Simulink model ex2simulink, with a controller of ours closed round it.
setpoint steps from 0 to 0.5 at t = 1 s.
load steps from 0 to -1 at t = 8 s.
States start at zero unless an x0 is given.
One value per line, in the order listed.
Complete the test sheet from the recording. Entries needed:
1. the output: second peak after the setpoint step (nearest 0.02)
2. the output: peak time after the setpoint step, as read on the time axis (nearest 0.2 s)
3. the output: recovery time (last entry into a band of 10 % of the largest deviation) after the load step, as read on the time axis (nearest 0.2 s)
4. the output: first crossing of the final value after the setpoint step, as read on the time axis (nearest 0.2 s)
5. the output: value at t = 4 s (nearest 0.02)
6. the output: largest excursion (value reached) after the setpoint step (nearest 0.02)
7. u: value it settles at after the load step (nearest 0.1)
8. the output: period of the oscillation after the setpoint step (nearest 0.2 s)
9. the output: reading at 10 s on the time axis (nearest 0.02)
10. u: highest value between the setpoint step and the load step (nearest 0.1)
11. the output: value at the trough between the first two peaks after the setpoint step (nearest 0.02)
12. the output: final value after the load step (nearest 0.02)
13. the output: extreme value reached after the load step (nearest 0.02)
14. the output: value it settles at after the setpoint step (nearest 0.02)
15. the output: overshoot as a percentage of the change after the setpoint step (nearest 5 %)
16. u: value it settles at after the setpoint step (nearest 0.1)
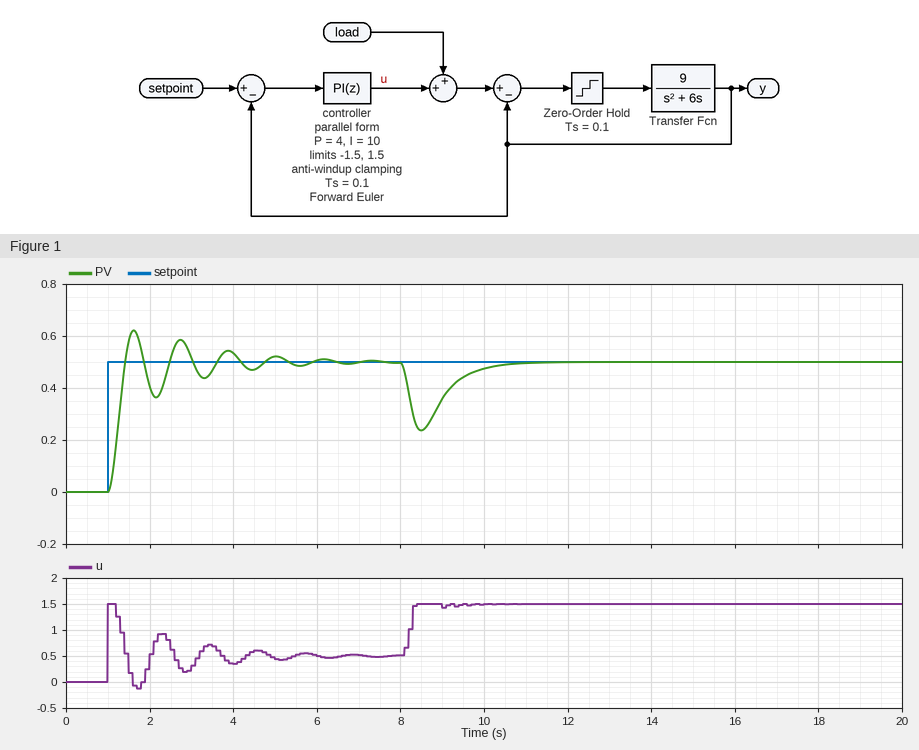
0.58
1.6 s
10.0 s
1.4 s
0.54
0.62
1.5
1.2 s
0.48
1.5
0.36
0.50
0.24
0.50
25 %
0.5
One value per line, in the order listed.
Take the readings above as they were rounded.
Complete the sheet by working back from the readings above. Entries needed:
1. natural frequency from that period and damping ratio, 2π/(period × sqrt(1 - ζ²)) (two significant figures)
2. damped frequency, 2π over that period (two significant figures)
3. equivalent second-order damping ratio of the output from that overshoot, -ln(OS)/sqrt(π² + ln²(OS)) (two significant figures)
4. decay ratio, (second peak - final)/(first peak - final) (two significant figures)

5.7 rad/s
5.2 rad/s
0.40
0.67
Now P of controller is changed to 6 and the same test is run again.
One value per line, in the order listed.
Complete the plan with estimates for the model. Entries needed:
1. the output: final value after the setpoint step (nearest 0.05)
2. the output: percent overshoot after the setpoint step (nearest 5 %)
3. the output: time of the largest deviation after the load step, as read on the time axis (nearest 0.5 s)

0.50
20 %
8.5 s
